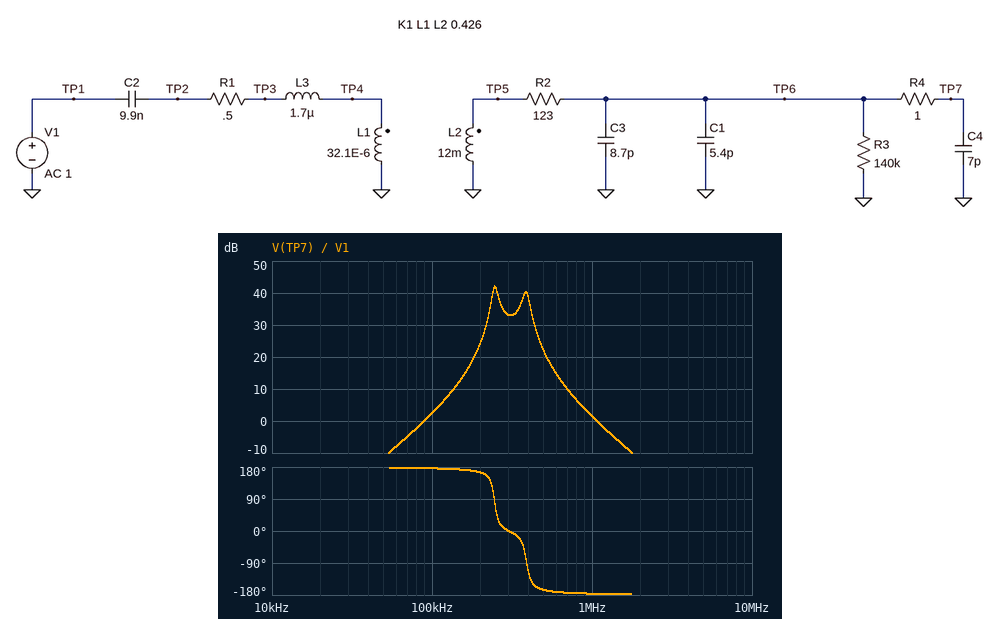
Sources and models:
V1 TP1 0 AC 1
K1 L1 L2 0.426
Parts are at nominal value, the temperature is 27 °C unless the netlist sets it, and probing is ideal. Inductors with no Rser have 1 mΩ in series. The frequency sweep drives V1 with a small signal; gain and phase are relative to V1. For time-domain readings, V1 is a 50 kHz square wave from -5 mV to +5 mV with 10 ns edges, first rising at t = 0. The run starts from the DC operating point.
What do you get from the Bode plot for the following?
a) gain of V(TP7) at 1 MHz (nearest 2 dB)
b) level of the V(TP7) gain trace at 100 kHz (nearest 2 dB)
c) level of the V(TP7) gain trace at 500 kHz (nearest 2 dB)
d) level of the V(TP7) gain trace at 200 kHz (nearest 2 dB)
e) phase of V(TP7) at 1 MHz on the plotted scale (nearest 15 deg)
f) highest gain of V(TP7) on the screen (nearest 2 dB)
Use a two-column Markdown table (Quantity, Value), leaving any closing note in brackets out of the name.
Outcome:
| Quantity | Value |
|---|---|
| gain of V(TP7) at 1 MHz | 2 dB |
| level of the V(TP7) gain trace at 100 kHz | 2 dB |
| level of the V(TP7) gain trace at 500 kHz | 22 dB |
| level of the V(TP7) gain trace at 200 kHz | 24 dB |
| phase of V(TP7) at 1 MHz on the plotted scale | -180 deg |
| highest gain of V(TP7) on the screen | 42 dB |
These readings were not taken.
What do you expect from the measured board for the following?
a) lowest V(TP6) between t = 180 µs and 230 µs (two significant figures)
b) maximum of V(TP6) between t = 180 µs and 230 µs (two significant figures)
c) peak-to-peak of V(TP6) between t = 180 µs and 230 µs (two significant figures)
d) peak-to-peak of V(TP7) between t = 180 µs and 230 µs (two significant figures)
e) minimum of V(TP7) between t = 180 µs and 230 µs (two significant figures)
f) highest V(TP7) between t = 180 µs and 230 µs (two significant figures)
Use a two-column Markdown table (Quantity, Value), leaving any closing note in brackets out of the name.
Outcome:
| Quantity | Value |
|---|---|
| lowest V(TP6) between t = 180 µs and 230 µs | -230 mV |
| maximum of V(TP6) between t = 180 µs and 230 µs | 230 mV |
| peak-to-peak of V(TP6) between t = 180 µs and 230 µs | 470 mV |
| peak-to-peak of V(TP7) between t = 180 µs and 230 µs | 470 mV |
| minimum of V(TP7) between t = 180 µs and 230 µs | -230 mV |
| highest V(TP7) between t = 180 µs and 230 µs | 230 mV |
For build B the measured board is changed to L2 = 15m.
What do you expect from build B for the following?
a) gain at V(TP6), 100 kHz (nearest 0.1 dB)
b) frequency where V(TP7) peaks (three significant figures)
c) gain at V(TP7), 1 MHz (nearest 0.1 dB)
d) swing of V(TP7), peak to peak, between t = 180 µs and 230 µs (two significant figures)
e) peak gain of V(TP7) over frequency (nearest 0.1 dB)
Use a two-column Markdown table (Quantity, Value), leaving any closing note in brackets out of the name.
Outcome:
| Quantity | Value |
|---|---|
| gain at V(TP6), 100 kHz | 3.6 dB |
| frequency where V(TP7) peaks | 362 kHz |
| gain at V(TP7), 1 MHz | 0.3 dB |
| swing of V(TP7), peak to peak, between t = 180 µs and 230 µs | 430 mV |
| peak gain of V(TP7) over frequency | 42.0 dB |
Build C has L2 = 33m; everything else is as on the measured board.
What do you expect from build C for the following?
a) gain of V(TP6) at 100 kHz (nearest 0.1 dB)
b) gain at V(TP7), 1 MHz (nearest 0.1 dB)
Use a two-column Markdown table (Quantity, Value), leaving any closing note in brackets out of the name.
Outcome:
| Quantity | Value |
|---|---|
| gain of V(TP6) at 100 kHz | 8.6 dB |
| gain at V(TP7), 1 MHz | -3.7 dB |
